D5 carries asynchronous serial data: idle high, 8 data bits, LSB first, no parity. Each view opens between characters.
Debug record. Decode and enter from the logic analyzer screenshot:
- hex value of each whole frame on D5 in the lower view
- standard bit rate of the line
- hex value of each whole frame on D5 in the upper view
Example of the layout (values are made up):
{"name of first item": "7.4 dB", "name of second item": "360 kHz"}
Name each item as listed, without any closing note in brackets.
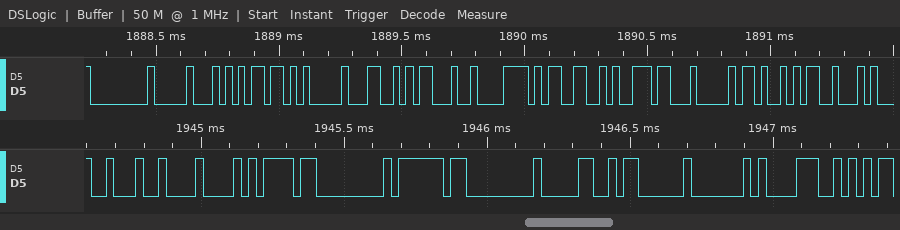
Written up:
{"hex value of each whole frame on D5 in the lower view": "22, 08, BD, 00, BF, 00, 30, 03, 40, 38", "standard bit rate of the line": "38400 baud", "hex value of each whole frame on D5 in the upper view": "00, 10, B5, 05, 4C, 23, 78, 33, B9, 04, 4B, 13"}
